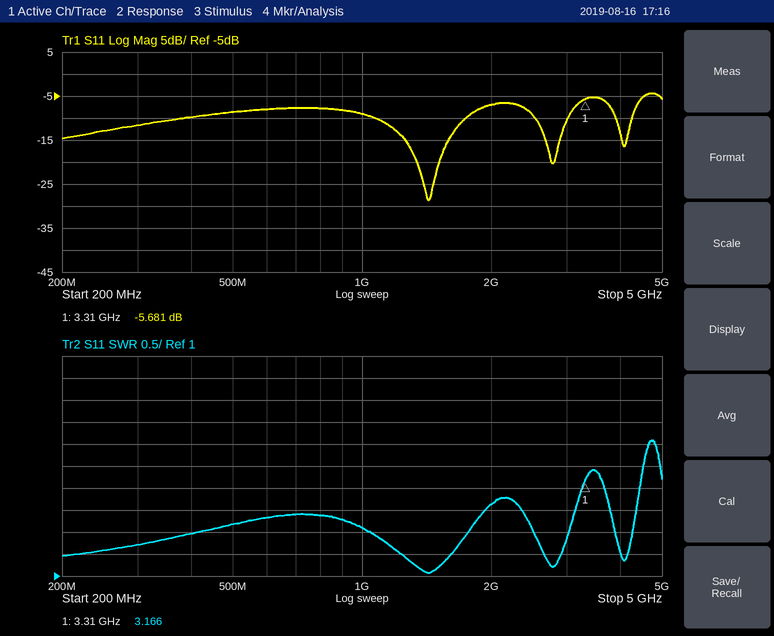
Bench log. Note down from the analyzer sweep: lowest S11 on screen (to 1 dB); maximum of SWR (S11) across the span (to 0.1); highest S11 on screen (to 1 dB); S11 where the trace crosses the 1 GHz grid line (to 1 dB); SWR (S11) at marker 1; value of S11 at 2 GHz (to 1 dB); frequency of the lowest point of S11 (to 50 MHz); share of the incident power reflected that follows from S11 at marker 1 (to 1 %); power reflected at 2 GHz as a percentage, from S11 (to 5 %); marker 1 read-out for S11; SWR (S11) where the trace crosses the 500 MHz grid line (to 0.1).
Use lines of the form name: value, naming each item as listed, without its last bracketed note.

lowest S11 on screen: -29 dB
maximum of SWR (S11) across the span: 4.1
highest S11 on screen: -4 dB
S11 where the trace crosses the 1 GHz grid line: -9 dB
SWR (S11) at marker 1: 3.166
value of S11 at 2 GHz: -7 dB
frequency of the lowest point of S11: 1.45 GHz
share of the incident power reflected that follows from S11 at marker 1: 27 %
power reflected at 2 GHz as a percentage, from S11: 20 %
marker 1 read-out for S11: -5.681 dB
SWR (S11) where the trace crosses the 500 MHz grid line: 2.2
